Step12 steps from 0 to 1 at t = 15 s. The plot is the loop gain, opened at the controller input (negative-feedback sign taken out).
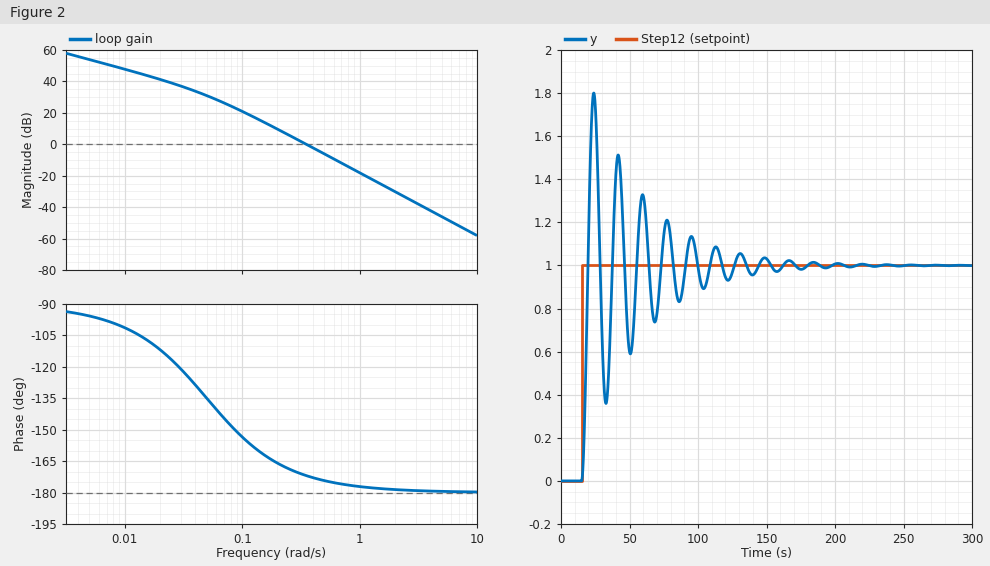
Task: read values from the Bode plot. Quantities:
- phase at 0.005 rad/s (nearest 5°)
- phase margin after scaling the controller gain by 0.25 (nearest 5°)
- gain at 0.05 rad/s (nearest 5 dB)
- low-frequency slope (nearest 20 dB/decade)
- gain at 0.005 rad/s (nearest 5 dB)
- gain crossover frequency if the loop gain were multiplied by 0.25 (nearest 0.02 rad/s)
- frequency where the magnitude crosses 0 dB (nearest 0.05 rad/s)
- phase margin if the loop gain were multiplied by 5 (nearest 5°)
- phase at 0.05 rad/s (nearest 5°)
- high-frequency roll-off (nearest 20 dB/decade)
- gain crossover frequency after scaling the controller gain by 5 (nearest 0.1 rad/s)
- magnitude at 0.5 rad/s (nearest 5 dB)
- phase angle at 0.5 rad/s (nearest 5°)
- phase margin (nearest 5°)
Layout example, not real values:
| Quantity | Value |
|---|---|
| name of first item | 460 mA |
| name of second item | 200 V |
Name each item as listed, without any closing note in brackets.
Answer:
| Quantity | Value |
|---|---|
| phase at 0.005 rad/s | -95° |
| phase margin after scaling the controller gain by 0.25 | 15° |
| gain at 0.05 rad/s | 30 dB |
| low-frequency slope | -20 dB/decade |
| gain at 0.005 rad/s | 55 dB |
| gain crossover frequency if the loop gain were multiplied by 0.25 | 0.18 rad/s |
| frequency where the magnitude crosses 0 dB | 0.35 rad/s |
| phase margin if the loop gain were multiplied by 5 | 5° |
| phase at 0.05 rad/s | -135° |
| high-frequency roll-off | -40 dB/decade |
| gain crossover frequency after scaling the controller gain by 5 | 0.8 rad/s |
| magnitude at 0.5 rad/s | -5 dB |
| phase angle at 0.5 rad/s | -175° |
| phase margin | 10° |
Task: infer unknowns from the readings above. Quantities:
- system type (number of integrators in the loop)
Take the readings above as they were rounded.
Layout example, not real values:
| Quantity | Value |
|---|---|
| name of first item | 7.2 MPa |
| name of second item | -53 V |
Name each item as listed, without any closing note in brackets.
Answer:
| Quantity | Value |
|---|---|
| system type | 1 |
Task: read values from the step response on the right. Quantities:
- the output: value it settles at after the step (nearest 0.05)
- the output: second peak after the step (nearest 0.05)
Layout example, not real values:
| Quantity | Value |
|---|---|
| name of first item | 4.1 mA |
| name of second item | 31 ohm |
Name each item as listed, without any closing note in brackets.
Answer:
| Quantity | Value |
|---|---|
| the output: value it settles at after the step | 1.00 |
| the output: second peak after the step | 1.50 |
